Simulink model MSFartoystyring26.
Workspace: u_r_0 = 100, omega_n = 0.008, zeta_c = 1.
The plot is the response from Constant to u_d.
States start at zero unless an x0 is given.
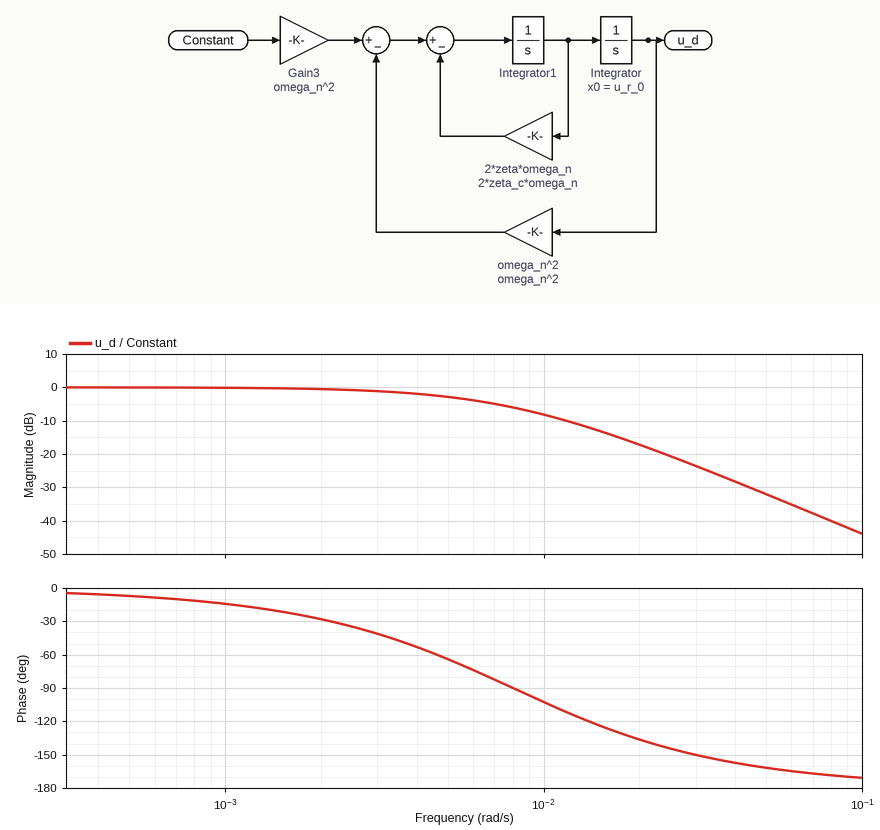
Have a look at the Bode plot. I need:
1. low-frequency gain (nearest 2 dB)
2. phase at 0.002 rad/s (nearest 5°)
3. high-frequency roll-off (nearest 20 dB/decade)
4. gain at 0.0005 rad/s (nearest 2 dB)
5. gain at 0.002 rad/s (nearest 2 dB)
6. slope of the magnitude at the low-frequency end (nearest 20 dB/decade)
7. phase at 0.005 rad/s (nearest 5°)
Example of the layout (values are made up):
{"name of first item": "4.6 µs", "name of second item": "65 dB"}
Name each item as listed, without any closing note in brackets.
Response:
{"low-frequency gain": "0 dB", "phase at 0.002 rad/s": "-30°", "high-frequency roll-off": "-40 dB/decade", "gain at 0.0005 rad/s": "0 dB", "gain at 0.002 rad/s": "0 dB", "slope of the magnitude at the low-frequency end": "0 dB/decade", "phase at 0.005 rad/s": "-65°"}
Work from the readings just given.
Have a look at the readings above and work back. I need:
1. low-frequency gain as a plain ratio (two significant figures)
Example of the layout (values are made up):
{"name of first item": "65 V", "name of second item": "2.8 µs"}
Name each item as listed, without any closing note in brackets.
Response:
{"low-frequency gain as a plain ratio": "1.0"}
